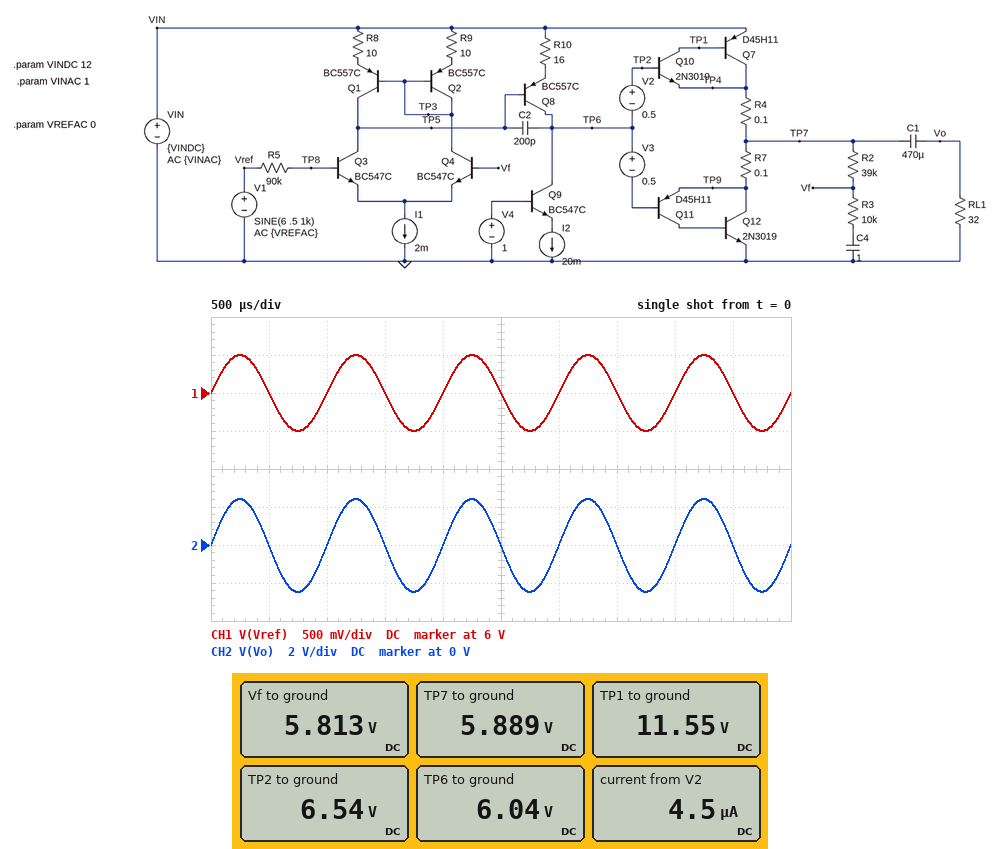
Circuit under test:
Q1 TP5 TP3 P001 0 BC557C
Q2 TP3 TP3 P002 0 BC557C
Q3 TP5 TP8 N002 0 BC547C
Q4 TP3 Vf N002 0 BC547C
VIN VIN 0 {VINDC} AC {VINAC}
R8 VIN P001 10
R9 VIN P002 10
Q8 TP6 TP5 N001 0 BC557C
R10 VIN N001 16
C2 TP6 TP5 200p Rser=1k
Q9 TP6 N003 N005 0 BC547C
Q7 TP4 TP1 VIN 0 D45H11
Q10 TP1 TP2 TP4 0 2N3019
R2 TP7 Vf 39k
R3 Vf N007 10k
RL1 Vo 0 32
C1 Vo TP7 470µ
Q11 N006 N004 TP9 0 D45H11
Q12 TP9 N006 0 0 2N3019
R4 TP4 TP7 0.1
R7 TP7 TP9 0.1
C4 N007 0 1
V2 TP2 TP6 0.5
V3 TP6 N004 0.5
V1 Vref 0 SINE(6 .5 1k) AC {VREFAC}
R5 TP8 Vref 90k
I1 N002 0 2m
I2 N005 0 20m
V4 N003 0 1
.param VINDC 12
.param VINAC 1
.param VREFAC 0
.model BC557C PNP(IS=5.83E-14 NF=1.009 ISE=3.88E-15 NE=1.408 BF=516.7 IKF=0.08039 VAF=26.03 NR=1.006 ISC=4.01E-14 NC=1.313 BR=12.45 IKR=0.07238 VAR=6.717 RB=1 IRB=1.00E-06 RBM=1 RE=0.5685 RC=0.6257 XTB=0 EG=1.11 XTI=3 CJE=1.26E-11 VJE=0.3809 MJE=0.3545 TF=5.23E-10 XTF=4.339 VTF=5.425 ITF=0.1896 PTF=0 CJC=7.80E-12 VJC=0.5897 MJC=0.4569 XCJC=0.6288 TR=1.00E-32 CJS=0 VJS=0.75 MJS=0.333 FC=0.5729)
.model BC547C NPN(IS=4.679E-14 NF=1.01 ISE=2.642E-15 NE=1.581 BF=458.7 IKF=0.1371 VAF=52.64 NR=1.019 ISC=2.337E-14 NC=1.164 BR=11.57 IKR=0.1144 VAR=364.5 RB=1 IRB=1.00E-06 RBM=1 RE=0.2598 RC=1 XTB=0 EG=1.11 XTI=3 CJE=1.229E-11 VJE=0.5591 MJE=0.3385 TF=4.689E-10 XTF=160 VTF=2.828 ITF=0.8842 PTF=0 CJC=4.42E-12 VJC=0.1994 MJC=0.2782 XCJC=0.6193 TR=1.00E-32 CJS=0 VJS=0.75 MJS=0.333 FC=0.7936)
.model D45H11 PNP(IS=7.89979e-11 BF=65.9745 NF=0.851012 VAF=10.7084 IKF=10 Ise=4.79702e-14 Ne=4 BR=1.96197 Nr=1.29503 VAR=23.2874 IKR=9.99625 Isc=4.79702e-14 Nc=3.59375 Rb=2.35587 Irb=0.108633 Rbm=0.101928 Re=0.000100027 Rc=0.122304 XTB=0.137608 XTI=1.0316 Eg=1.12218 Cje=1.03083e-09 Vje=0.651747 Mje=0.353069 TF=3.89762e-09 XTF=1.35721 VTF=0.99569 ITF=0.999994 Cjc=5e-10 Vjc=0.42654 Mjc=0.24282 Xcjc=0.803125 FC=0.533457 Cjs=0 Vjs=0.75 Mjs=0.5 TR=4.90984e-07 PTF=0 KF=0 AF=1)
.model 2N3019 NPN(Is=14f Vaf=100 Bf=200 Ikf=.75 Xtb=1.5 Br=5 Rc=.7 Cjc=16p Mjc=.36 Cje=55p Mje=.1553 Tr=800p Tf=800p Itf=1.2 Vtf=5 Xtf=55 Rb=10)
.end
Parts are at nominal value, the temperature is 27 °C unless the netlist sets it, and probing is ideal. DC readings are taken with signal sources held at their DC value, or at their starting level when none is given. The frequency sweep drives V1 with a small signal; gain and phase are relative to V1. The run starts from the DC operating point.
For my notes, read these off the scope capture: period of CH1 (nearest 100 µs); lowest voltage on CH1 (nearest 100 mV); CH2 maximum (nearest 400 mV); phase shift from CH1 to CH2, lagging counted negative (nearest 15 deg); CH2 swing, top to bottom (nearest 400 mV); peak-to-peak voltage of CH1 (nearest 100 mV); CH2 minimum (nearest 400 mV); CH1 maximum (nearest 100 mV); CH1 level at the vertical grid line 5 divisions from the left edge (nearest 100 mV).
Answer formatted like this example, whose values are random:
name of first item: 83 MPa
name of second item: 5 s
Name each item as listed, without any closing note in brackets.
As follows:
period of CH1: 1.0 ms
lowest voltage on CH1: 5.5 V
CH2 maximum: 2.4 V
phase shift from CH1 to CH2, lagging counted negative: 0 deg
CH2 swing, top to bottom: 4.8 V
peak-to-peak voltage of CH1: 1.0 V
CH2 minimum: -2.4 V
CH1 maximum: 6.5 V
CH1 level at the vertical grid line 5 divisions from the left edge: 6.0 V
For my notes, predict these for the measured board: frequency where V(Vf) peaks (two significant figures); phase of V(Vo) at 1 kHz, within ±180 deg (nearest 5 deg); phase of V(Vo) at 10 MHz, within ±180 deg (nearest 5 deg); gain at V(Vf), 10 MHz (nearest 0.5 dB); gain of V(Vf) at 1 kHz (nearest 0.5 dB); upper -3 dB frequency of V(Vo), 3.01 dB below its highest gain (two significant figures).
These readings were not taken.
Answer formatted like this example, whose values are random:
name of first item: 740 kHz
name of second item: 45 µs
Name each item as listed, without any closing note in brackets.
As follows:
frequency where V(Vf) peaks: 4.7 MHz
phase of V(Vo) at 1 kHz, within ±180 deg: 0 deg
phase of V(Vo) at 10 MHz, within ±180 deg: 55 deg
gain at V(Vf), 10 MHz: -1.5 dB
gain of V(Vf) at 1 kHz: 0 dB
upper -3 dB frequency of V(Vo), 3.01 dB below its highest gain: 5.0 MHz
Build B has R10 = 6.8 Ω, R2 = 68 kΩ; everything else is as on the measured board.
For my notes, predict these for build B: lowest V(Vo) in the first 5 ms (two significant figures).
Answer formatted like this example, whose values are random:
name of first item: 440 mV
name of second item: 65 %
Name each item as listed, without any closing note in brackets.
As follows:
lowest V(Vo) in the first 5 ms: -3.9 V
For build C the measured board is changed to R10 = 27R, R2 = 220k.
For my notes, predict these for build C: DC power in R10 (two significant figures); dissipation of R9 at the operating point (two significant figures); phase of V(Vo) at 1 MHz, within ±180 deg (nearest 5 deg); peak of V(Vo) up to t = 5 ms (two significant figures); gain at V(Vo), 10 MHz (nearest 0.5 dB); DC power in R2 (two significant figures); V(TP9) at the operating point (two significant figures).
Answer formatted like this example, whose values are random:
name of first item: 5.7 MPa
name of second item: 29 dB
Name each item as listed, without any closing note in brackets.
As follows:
DC power in R10: 11 mW
dissipation of R9 at the operating point: 9.3 µW
phase of V(Vo) at 1 MHz, within ±180 deg: -75 deg
peak of V(Vo) up to t = 5 ms: 5.0 V
gain at V(Vo), 10 MHz: -9.5 dB
DC power in R2: 820 nW
V(TP9) at the operating point: 6.2 V
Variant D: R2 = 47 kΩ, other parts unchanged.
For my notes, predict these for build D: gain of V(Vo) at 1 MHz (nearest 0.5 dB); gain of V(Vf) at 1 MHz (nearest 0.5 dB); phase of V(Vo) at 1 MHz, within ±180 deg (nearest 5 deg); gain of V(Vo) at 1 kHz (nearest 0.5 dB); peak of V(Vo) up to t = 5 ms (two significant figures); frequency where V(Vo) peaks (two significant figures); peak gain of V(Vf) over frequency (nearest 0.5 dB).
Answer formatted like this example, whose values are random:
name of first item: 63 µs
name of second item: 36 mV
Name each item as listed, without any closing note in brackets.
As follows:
gain of V(Vo) at 1 MHz: 10.5 dB
gain of V(Vf) at 1 MHz: -5.5 dB
phase of V(Vo) at 1 MHz, within ±180 deg: -45 deg
gain of V(Vo) at 1 kHz: 15.0 dB
peak of V(Vo) up to t = 5 ms: 2.8 V
frequency where V(Vo) peaks: 4.5 MHz
peak gain of V(Vf) over frequency: 0 dB
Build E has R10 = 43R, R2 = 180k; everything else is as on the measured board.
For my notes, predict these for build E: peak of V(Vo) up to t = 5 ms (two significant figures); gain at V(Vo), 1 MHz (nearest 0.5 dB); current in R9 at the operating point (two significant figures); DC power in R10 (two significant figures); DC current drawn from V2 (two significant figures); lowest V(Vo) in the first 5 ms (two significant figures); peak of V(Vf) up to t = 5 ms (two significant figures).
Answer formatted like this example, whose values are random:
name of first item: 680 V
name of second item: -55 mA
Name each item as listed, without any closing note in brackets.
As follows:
peak of V(Vo) up to t = 5 ms: 4.8 V
gain at V(Vo), 1 MHz: 11.0 dB
current in R9 at the operating point: 960 µA
DC power in R10: 17 mW
DC current drawn from V2: 4.6 µA
lowest V(Vo) in the first 5 ms: -5.7 V
peak of V(Vf) up to t = 5 ms: 6.1 V
